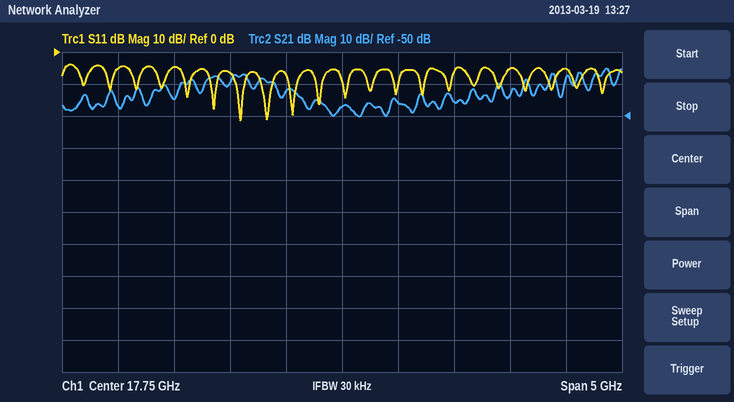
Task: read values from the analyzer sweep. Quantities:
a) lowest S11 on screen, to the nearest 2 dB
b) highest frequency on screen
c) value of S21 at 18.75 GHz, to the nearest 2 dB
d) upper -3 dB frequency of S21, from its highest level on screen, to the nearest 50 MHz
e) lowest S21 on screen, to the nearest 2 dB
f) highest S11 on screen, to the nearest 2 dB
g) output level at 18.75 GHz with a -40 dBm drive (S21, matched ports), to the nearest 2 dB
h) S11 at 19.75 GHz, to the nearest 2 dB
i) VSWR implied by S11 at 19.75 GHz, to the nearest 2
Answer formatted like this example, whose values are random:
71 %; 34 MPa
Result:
-22 dB; 20.25 GHz; -46 dB; 20.15 GHz; -50 dB; -4 dB; -86 dBm; -6 dB; 4
